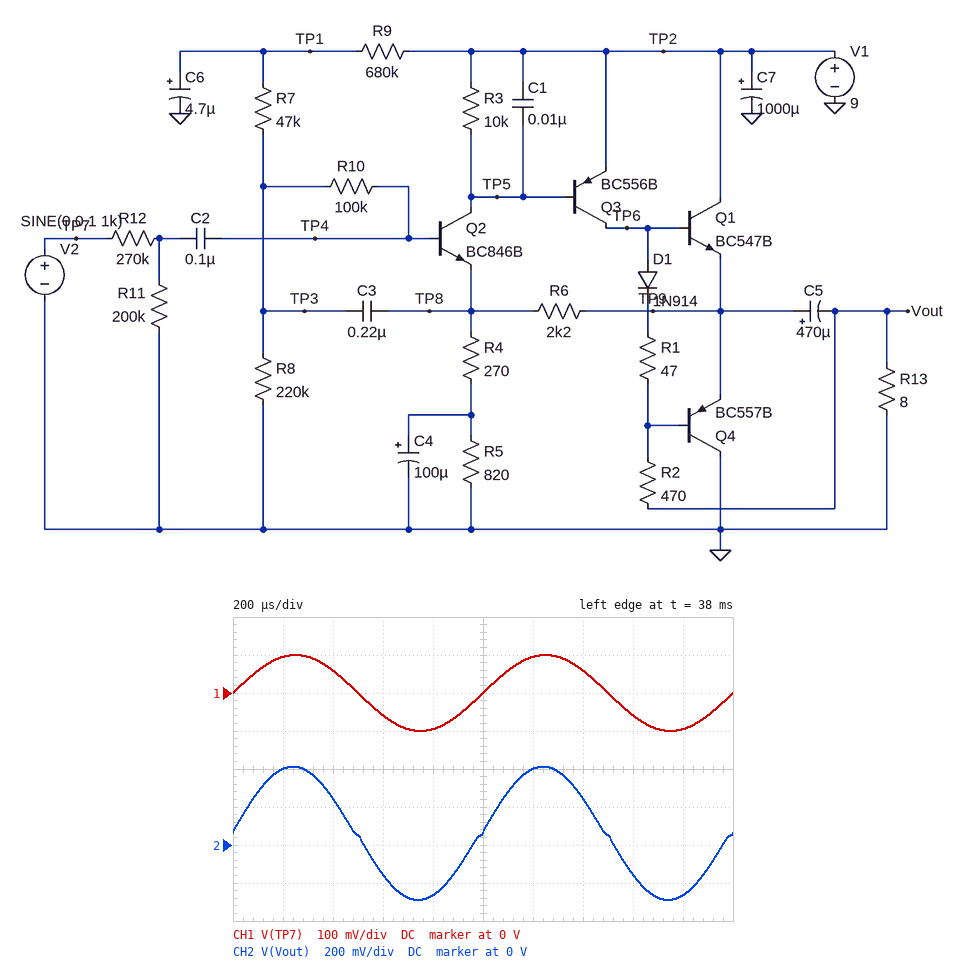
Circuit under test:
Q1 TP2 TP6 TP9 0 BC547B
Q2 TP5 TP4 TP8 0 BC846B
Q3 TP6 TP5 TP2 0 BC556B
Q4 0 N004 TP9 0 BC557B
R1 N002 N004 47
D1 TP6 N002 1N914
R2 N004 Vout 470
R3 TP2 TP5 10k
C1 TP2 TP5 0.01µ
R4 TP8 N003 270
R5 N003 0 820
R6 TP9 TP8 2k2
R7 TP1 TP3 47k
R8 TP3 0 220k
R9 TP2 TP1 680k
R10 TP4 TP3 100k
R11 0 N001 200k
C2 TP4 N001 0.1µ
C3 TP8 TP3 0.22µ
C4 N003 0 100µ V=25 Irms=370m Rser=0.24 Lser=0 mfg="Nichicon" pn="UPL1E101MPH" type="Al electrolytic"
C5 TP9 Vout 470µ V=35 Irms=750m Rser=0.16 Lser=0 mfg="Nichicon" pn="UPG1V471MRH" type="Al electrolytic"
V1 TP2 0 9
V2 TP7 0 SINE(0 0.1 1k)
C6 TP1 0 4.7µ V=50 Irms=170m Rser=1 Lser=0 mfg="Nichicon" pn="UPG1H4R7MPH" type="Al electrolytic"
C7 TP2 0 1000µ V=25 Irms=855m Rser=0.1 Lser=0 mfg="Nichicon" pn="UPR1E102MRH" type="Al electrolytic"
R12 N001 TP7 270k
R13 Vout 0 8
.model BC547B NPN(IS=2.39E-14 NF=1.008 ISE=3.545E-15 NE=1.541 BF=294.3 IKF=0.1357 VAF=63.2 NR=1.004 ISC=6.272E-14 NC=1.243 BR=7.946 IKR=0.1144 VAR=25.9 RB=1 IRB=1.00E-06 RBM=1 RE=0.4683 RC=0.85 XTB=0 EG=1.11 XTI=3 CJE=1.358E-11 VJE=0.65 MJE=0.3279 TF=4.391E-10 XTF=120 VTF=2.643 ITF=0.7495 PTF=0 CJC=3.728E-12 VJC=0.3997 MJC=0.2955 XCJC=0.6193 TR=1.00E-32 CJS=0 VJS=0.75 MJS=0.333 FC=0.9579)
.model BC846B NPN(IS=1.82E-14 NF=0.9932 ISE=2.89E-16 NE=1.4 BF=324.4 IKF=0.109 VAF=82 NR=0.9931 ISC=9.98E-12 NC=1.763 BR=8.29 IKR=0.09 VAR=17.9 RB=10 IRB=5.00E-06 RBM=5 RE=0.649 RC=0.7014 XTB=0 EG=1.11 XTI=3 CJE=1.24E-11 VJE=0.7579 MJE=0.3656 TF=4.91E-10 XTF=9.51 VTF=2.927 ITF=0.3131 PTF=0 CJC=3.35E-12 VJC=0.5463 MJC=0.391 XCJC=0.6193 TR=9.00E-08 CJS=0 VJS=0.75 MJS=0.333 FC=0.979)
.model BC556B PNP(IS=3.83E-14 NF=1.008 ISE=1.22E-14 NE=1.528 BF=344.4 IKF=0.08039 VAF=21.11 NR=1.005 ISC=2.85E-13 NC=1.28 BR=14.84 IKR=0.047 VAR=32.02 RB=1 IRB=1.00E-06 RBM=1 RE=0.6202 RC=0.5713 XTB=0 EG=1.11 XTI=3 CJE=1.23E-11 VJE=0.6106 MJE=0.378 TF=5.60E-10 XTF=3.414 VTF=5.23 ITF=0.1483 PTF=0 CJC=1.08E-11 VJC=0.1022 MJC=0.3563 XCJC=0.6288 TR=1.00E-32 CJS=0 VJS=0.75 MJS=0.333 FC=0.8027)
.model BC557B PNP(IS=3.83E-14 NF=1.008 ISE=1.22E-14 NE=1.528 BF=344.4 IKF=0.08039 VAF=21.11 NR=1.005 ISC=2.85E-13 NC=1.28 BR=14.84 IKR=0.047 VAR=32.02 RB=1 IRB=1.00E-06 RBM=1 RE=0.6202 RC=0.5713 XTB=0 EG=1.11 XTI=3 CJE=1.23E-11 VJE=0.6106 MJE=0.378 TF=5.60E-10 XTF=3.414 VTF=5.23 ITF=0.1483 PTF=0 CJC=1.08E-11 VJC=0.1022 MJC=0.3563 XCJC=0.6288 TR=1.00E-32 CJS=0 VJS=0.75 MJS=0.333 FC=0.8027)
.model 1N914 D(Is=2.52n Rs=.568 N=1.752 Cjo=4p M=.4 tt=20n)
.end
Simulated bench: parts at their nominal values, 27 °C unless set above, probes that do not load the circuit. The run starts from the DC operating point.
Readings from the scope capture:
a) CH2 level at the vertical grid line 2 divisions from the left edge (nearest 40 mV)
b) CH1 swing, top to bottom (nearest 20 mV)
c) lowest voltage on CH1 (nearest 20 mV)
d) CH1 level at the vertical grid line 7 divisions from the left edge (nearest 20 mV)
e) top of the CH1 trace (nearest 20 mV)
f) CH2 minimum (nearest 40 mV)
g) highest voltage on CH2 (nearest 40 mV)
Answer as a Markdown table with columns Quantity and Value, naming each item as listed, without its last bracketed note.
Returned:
| Quantity | Value |
|---|---|
| CH2 level at the vertical grid line 2 divisions from the left edge | 240 mV |
| CH1 swing, top to bottom | 200 mV |
| lowest voltage on CH1 | -100 mV |
| CH1 level at the vertical grid line 7 divisions from the left edge | 60 mV |
| top of the CH1 trace | 100 mV |
| CH2 minimum | -280 mV |
| highest voltage on CH2 | 400 mV |
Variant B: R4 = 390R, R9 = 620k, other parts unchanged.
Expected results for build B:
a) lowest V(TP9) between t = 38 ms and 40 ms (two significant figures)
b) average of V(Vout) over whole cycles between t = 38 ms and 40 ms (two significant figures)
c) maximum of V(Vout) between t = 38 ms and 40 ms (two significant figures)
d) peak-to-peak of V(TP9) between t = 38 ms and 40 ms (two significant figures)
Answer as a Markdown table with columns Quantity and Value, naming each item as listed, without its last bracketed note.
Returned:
| Quantity | Value |
|---|---|
| lowest V(TP9) between t = 38 ms and 40 ms | 4.0 V |
| average of V(Vout) over whole cycles between t = 38 ms and 40 ms | 63 mV |
| maximum of V(Vout) between t = 38 ms and 40 ms | 320 mV |
| peak-to-peak of V(TP9) between t = 38 ms and 40 ms | 530 mV |
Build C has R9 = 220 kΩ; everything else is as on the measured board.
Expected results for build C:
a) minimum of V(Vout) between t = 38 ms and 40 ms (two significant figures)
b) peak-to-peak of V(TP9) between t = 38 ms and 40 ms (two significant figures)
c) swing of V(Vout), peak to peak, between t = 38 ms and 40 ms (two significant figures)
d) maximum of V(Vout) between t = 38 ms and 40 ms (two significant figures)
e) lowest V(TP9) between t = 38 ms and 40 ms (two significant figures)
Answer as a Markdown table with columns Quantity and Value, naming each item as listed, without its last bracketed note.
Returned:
| Quantity | Value |
|---|---|
| minimum of V(Vout) between t = 38 ms and 40 ms | 120 mV |
| peak-to-peak of V(TP9) between t = 38 ms and 40 ms | 5.9 mV |
| swing of V(Vout), peak to peak, between t = 38 ms and 40 ms | 5.7 mV |
| maximum of V(Vout) between t = 38 ms and 40 ms | 130 mV |
| lowest V(TP9) between t = 38 ms and 40 ms | 8.2 V |
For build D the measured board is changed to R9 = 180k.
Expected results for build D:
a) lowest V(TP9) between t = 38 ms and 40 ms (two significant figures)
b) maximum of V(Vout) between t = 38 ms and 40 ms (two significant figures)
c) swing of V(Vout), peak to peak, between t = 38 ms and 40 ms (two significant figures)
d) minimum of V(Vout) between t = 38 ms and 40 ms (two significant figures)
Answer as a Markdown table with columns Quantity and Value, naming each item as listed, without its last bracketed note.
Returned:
| Quantity | Value |
|---|---|
| lowest V(TP9) between t = 38 ms and 40 ms | 8.2 V |
| maximum of V(Vout) between t = 38 ms and 40 ms | 130 mV |
| swing of V(Vout), peak to peak, between t = 38 ms and 40 ms | 3.1 mV |
| minimum of V(Vout) between t = 38 ms and 40 ms | 120 mV |
